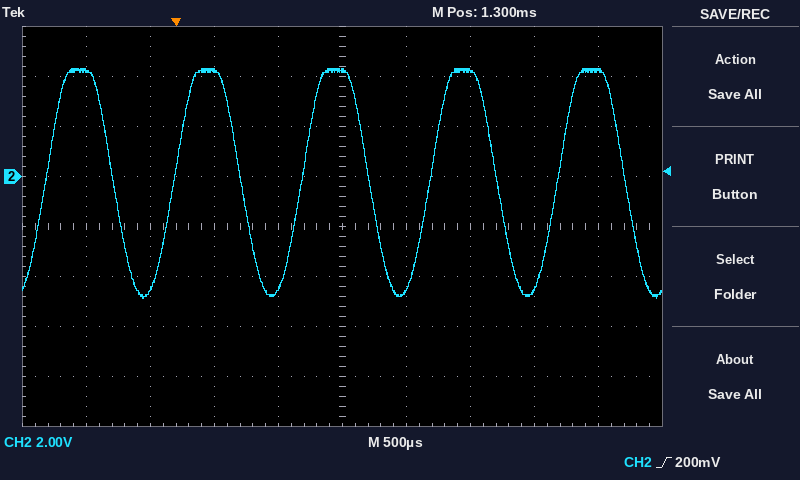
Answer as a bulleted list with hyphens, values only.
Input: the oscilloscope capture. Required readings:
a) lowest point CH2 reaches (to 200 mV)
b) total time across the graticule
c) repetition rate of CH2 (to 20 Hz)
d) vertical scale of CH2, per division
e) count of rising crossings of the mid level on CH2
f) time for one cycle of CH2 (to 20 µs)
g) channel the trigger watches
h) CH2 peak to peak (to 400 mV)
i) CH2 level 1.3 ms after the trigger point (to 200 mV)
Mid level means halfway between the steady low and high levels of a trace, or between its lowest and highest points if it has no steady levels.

- -4.8 V
- 5 ms
- 1.00 kHz
- 2 V
- 5
- 1.00 ms
- CH2
- 9.2 V
- 4.2 V
